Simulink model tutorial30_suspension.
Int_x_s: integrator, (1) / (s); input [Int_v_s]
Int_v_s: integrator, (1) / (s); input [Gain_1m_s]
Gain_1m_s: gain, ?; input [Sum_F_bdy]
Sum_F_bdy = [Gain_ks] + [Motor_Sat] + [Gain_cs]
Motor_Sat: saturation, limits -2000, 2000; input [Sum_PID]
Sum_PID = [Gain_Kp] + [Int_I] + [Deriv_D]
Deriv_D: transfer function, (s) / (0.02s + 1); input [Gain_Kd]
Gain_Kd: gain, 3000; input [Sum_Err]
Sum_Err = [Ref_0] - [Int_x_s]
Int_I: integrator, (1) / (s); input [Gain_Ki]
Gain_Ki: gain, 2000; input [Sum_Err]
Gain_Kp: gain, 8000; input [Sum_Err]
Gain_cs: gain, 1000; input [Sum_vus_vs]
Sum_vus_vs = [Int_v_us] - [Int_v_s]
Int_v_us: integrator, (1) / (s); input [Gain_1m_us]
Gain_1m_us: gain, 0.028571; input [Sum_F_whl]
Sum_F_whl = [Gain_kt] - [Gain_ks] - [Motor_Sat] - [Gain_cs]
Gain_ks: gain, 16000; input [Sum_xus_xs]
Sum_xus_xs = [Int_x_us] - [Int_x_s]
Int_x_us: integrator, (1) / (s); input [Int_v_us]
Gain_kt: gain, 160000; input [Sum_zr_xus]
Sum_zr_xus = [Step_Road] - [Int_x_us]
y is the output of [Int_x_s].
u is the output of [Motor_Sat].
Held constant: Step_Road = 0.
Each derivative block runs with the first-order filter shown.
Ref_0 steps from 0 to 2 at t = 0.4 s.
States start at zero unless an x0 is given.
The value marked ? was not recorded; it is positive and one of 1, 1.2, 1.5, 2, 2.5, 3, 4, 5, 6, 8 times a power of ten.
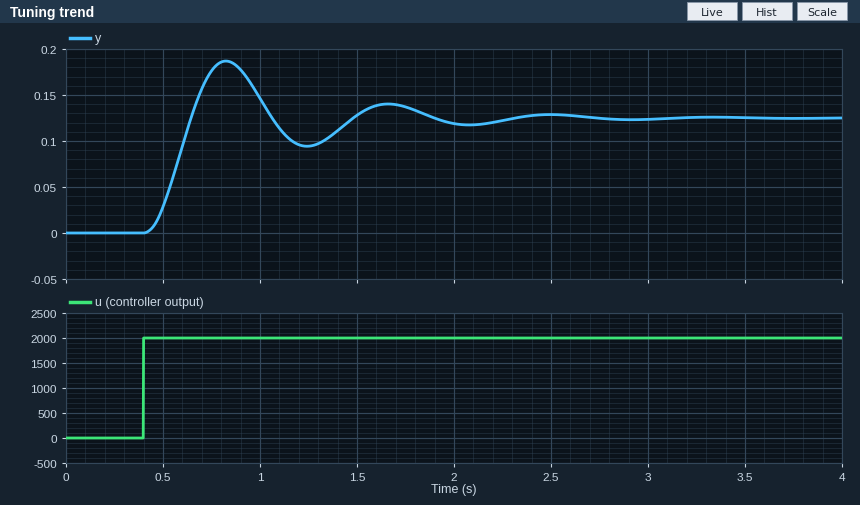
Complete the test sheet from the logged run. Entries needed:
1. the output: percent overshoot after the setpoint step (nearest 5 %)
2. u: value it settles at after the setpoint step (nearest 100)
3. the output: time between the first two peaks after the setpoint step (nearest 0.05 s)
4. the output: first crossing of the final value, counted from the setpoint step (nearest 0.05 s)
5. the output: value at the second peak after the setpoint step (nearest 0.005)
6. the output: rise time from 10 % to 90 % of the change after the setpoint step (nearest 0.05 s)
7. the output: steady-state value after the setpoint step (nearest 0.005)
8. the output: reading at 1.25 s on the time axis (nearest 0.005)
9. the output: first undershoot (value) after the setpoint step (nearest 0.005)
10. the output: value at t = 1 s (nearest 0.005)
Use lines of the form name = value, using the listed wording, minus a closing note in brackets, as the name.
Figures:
the output: percent overshoot after the setpoint step = 50 %
u: value it settles at after the setpoint step = 2000
the output: time between the first two peaks after the setpoint step = 0.85 s
the output: first crossing of the final value, counted from the setpoint step = 0.25 s
the output: value at the second peak after the setpoint step = 0.140
the output: rise time from 10 % to 90 % of the change after the setpoint step = 0.15 s
the output: steady-state value after the setpoint step = 0.125
the output: reading at 1.25 s on the time axis = 0.095
the output: first undershoot (value) after the setpoint step = 0.095
the output: value at t = 1 s = 0.145
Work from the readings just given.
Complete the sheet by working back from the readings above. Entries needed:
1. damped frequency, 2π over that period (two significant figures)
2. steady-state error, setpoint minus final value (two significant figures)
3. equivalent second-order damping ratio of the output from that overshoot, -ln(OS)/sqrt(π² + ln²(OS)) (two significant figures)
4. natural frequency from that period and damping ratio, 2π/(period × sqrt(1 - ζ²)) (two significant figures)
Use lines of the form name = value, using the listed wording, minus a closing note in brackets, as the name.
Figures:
damped frequency, 2π over that period = 7.4 rad/s
steady-state error, setpoint minus final value = 1.9
equivalent second-order damping ratio of the output from that overshoot, -ln(OS)/sqrt(π² + ln²(OS)) = 0.22
natural frequency from that period and damping ratio, 2π/(period × sqrt(1 - ζ²)) = 7.6 rad/s
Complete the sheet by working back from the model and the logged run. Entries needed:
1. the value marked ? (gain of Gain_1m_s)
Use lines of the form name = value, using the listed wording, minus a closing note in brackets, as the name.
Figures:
the value marked ? = 0.004
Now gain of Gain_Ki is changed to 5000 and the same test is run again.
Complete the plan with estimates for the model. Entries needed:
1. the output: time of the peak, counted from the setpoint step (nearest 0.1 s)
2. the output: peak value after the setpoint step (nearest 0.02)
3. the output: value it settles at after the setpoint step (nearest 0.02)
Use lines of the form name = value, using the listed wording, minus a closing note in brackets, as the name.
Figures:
the output: time of the peak, counted from the setpoint step = 0.4 s
the output: peak value after the setpoint step = 0.18
the output: value it settles at after the setpoint step = 0.12
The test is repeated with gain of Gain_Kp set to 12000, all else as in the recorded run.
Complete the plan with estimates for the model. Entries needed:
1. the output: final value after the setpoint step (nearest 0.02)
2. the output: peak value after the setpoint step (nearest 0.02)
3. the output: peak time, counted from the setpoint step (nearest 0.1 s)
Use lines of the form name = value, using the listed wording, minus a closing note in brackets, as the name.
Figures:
the output: final value after the setpoint step = 0.12
the output: peak value after the setpoint step = 0.18
the output: peak time, counted from the setpoint step = 0.4 s
